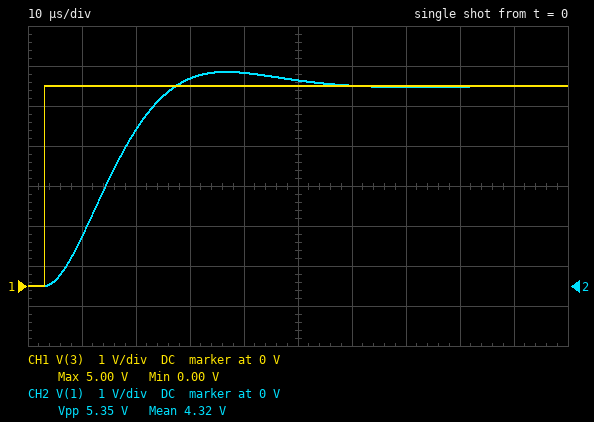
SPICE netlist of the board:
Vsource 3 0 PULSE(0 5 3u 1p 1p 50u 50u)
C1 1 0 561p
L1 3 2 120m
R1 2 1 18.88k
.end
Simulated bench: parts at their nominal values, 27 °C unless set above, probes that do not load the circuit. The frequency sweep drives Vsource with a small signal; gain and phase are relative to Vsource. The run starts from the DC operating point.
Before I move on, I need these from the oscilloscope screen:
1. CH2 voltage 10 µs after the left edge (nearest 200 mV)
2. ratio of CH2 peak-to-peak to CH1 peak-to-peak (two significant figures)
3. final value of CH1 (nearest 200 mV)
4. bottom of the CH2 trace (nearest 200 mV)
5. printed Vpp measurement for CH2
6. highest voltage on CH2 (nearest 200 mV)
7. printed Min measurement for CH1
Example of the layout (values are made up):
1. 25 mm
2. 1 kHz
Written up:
1. 1.2 V
2. 1.1
3. 5.0 V
4. 0 V
5. 5.35 V
6. 5.4 V
7. 0.00 V
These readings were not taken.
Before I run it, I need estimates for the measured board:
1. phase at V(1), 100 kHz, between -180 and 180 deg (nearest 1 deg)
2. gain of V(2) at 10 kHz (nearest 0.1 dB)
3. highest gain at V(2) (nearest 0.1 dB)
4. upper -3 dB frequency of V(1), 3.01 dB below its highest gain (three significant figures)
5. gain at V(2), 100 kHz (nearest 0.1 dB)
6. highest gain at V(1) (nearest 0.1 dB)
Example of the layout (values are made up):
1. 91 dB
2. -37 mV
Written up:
1. -165 deg
2. 1.7 dB
3. 2.4 dB
4. 20.8 kHz
5. -11.9 dB
6. 0.1 dB
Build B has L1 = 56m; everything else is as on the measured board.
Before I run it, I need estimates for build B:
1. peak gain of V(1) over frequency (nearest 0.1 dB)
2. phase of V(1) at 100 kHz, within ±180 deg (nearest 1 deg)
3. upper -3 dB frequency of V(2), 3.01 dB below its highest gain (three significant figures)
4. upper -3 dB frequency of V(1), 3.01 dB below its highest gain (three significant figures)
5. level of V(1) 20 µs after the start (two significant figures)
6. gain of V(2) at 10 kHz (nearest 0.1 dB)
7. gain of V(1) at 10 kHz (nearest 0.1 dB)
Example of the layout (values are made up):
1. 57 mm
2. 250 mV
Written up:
1. 0 dB
2. -150 deg
3. 55.1 kHz
4. 19.8 kHz
5. 4.2 V
6. 0.8 dB
7. -0.8 dB
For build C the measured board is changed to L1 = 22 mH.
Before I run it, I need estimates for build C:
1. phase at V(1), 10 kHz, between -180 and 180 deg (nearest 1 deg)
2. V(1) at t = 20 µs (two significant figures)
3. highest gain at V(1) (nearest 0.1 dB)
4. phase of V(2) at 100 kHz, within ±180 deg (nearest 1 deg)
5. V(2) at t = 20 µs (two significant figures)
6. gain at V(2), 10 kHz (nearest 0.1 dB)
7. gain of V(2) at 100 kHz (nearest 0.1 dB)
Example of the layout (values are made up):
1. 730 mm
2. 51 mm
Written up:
1. -35 deg
2. 4.1 V
3. 0 dB
4. -39 deg
5. 5.1 V
6. 0.3 dB
7. -1.2 dB
